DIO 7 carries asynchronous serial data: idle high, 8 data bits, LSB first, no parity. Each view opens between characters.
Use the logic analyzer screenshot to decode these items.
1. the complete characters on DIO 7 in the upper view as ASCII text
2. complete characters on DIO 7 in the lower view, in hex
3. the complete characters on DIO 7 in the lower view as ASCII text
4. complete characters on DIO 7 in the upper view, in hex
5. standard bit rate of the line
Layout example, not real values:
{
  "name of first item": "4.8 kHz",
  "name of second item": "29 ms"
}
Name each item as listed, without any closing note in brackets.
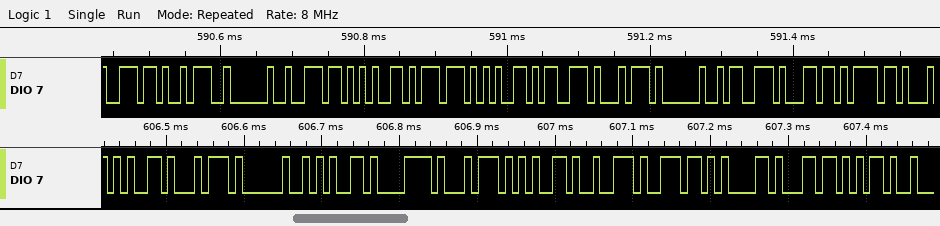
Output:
{
  "the complete characters on DIO 7 in the upper view as ASCII text": "\"n: newest slo\"",
  "complete characters on DIO 7 in the lower view, in hex": "65, 74, 20, 65, 78, 74, 65, 72, 6E, 61, 6C, 2D",
  "the complete characters on DIO 7 in the lower view as ASCII text": "\"et external-\"",
  "complete characters on DIO 7 in the upper view, in hex": "6E, 3A, 20, 6E, 65, 77, 65, 73, 74, 20, 73, 6C, 6F",
  "standard bit rate of the line": "115200 baud"
}
